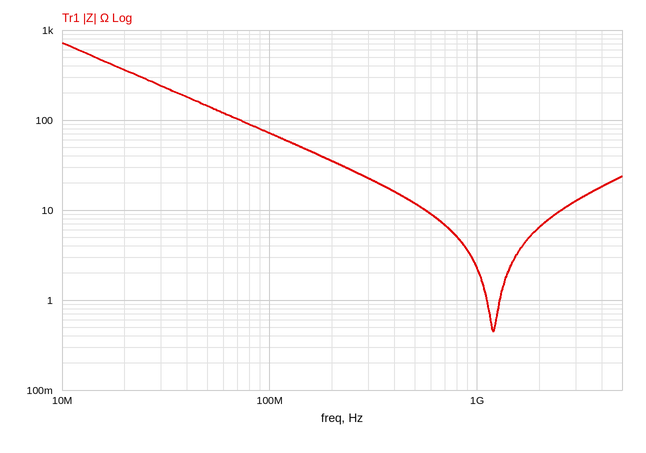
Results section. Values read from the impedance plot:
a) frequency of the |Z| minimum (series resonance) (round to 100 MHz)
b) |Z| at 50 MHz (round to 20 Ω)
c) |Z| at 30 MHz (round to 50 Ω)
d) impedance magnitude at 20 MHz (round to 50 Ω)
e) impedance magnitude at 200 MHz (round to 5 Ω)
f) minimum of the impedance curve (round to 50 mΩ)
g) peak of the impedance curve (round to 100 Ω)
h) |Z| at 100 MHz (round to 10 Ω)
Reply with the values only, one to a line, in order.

1.2 GHz
140 Ω
250 Ω
350 Ω
35 Ω
450 mΩ
700 Ω
70 Ω
